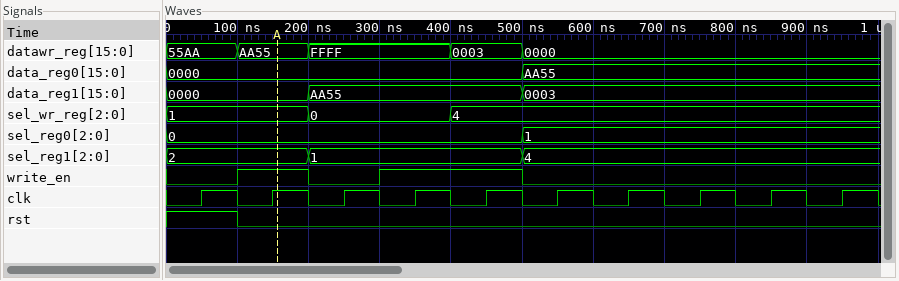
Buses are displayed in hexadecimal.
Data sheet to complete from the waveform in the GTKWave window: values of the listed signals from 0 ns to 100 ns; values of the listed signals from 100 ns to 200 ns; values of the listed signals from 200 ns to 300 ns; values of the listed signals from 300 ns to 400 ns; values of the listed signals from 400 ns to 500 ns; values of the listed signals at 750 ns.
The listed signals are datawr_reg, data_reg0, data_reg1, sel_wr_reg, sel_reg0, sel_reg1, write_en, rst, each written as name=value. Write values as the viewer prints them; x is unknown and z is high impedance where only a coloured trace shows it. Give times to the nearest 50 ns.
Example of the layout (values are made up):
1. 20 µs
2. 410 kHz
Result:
1. datawr_reg=55AA, data_reg0=0000, data_reg1=0000, sel_wr_reg=1, sel_reg0=0, sel_reg1=2, write_en=0, rst=1
2. datawr_reg=AA55, data_reg0=0000, data_reg1=0000, sel_wr_reg=1, sel_reg0=0, sel_reg1=2, write_en=1, rst=0
3. datawr_reg=FFFF, data_reg0=0000, data_reg1=AA55, sel_wr_reg=0, sel_reg0=0, sel_reg1=1, write_en=0, rst=0
4. datawr_reg=FFFF, data_reg0=0000, data_reg1=AA55, sel_wr_reg=0, sel_reg0=0, sel_reg1=1, write_en=1, rst=0
5. datawr_reg=0003, data_reg0=0000, data_reg1=AA55, sel_wr_reg=4, sel_reg0=0, sel_reg1=1, write_en=1, rst=0
6. datawr_reg=0000, data_reg0=AA55, data_reg1=0003, sel_wr_reg=4, sel_reg0=1, sel_reg1=4, write_en=0, rst=0
